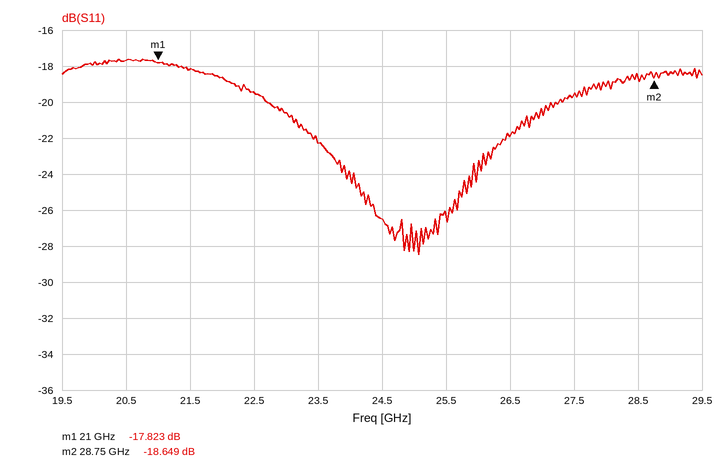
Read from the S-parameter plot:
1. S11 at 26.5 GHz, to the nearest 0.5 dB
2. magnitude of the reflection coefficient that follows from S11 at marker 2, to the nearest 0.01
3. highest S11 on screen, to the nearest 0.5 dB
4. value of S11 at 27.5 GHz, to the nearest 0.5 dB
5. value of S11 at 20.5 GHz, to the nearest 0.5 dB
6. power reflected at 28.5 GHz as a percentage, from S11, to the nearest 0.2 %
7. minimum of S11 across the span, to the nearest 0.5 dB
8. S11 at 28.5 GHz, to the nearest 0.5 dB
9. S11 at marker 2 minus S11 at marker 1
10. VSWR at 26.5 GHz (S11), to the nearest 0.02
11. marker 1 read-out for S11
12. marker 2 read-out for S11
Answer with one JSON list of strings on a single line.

["-22.0 dB", "0.12", "-17.5 dB", "-19.5 dB", "-17.5 dB", "1.4 %", "-28.5 dB", "-18.5 dB", "-0.826 dB", "1.18", "-17.823 dB", "-18.649 dB"]
